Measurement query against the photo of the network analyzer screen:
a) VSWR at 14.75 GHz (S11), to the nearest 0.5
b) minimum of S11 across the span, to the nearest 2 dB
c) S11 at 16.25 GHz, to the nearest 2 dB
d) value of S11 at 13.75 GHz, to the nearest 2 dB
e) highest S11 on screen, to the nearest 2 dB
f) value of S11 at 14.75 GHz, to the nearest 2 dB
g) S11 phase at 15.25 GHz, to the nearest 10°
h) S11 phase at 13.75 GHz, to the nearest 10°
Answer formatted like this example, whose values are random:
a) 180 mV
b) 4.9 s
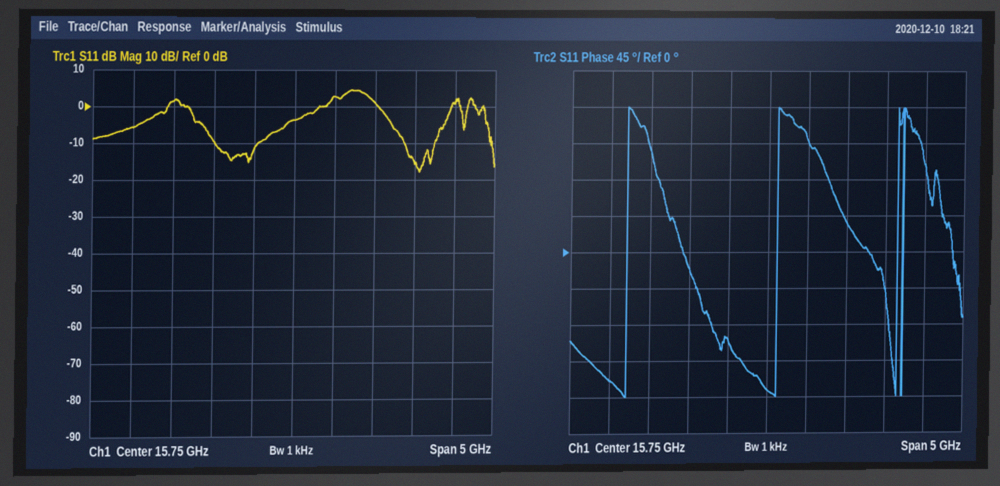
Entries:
a) 2.0
b) -18 dB
c) 2 dB
d) -6 dB
e) 4 dB
f) -10 dB
g) -110°
h) -160°
